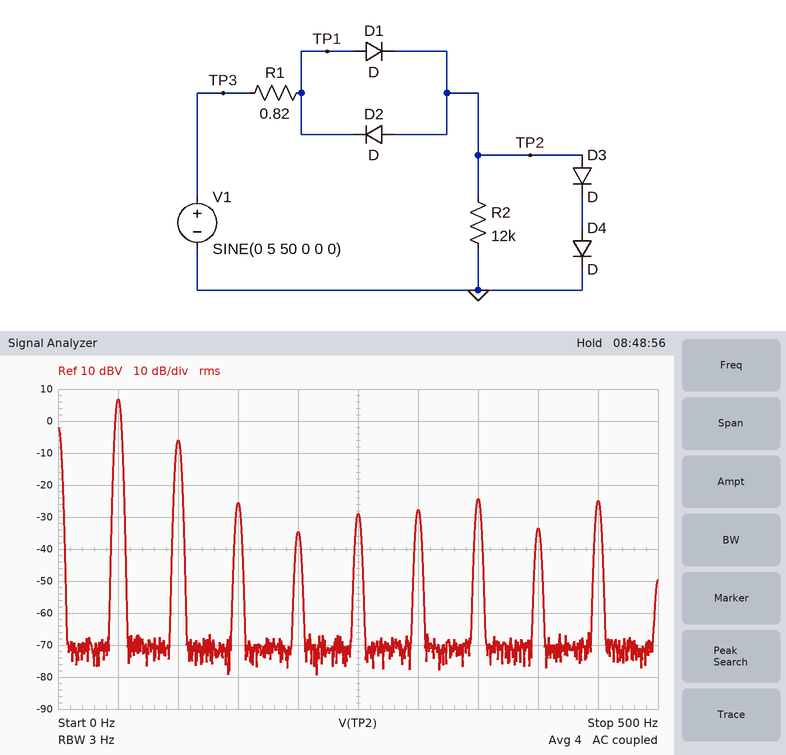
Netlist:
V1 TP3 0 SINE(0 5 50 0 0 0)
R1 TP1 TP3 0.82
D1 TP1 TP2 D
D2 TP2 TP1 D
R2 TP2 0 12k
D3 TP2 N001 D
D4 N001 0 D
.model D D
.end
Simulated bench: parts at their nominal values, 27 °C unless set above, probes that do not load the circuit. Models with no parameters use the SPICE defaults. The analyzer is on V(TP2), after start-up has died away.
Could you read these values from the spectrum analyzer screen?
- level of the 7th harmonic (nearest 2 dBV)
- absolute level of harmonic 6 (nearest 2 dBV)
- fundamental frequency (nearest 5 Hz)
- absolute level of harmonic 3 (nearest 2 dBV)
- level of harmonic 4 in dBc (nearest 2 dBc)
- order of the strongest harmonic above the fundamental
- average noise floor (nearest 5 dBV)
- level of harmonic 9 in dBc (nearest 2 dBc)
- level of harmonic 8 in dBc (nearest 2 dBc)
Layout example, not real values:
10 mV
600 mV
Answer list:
-24 dBV
-28 dBV
50 Hz
-26 dBV
-42 dBc
2
-70 dBV
-32 dBc
-40 dBc
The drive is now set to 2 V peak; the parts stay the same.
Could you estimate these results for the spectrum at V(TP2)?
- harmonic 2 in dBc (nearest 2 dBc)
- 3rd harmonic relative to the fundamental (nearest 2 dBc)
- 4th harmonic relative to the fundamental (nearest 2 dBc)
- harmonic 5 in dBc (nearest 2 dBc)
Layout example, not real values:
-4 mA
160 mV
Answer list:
-40 dBc
-16 dBc
-42 dBc
-22 dBc
